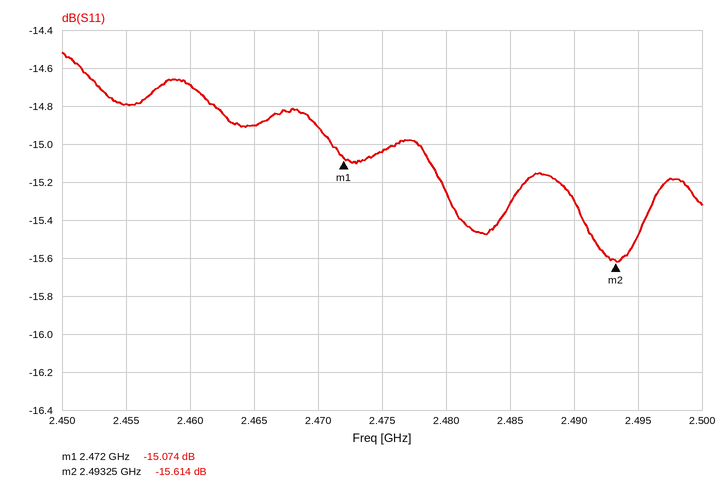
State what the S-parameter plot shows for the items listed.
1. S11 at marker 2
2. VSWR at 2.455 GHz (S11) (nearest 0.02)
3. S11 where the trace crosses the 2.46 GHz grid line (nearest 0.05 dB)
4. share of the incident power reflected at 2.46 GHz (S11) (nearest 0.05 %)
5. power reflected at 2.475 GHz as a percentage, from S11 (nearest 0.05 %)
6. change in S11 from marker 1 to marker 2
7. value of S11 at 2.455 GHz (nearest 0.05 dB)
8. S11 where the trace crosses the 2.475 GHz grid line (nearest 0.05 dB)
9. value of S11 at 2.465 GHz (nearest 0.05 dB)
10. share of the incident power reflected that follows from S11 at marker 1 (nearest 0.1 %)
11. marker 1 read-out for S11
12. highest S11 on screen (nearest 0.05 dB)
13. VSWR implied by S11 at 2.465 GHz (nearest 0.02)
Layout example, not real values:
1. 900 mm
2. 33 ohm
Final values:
1. -15.614 dB
2. 1.44
3. -14.70 dB
4. 3.40 %
5. 3.15 %
6. -0.540 dB
7. -14.80 dB
8. -15.05 dB
9. -14.90 dB
10. 3.1 %
11. -15.074 dB
12. -14.50 dB
13. 1.44
